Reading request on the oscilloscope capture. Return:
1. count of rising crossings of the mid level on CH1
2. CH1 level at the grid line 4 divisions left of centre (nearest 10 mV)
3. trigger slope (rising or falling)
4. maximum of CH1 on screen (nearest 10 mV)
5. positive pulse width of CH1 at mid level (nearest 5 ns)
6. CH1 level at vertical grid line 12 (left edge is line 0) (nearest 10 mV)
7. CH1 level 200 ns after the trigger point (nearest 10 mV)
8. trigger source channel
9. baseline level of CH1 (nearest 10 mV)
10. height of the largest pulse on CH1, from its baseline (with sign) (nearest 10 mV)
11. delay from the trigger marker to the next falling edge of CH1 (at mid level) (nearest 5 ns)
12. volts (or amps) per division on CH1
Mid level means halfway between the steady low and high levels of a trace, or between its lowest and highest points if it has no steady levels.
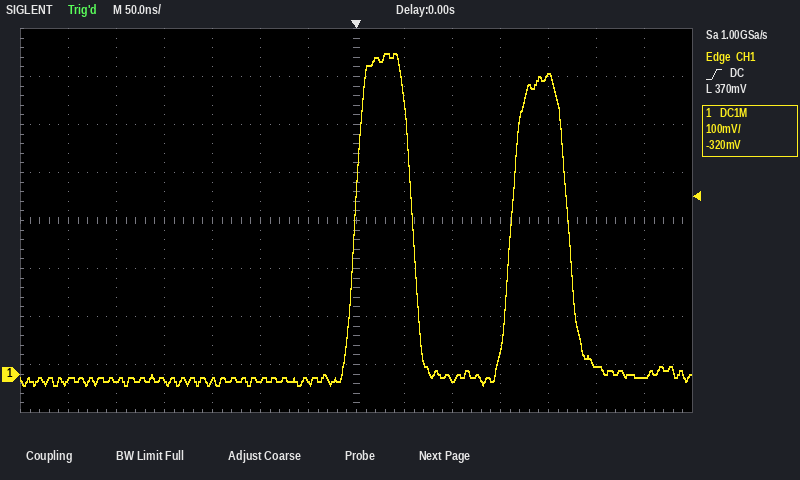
2
-10 mV
rising
670 mV
60 ns
20 mV
620 mV
CH1
-10 mV
+680 mV
60 ns
100 mV
